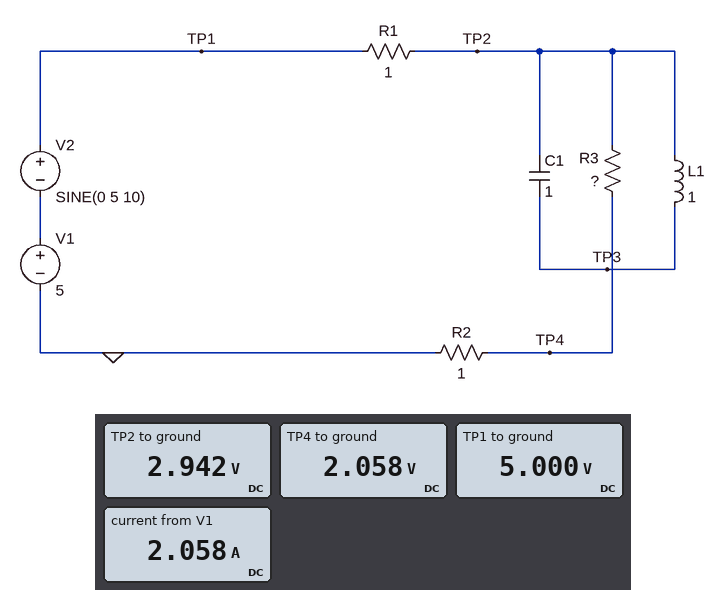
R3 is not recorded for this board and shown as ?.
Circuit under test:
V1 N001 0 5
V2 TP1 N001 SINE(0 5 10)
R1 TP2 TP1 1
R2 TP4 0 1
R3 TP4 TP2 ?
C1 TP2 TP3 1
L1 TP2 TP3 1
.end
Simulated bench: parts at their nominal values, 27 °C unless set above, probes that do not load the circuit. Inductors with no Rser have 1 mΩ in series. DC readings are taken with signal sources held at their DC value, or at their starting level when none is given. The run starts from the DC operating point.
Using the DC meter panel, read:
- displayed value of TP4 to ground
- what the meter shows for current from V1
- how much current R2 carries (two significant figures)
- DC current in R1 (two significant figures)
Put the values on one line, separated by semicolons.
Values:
2.058 V; 2.058 A; 2.1 A; 2.1 A
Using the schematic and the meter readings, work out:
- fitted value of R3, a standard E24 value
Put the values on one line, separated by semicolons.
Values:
0.43 Ω
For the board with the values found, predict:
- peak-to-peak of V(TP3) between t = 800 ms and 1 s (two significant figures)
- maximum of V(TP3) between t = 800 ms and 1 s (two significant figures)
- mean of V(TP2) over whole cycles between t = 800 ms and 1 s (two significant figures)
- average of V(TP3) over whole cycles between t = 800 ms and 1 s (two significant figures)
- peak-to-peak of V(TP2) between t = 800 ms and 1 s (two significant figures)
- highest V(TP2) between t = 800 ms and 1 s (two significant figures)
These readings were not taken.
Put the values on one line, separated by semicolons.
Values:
5.9 V; 5.9 V; 2.9 V; 2.9 V; 5.9 V; 5.9 V
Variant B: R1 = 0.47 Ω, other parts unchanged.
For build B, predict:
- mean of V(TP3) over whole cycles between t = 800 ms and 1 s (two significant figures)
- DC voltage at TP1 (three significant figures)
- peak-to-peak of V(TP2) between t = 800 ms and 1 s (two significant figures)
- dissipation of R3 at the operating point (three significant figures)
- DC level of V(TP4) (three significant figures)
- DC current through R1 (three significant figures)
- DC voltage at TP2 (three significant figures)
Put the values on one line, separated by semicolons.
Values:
3.8 V; 5.00 V; 7.5 V; 2.98 W; 2.63 V; 2.63 A; 3.76 V
